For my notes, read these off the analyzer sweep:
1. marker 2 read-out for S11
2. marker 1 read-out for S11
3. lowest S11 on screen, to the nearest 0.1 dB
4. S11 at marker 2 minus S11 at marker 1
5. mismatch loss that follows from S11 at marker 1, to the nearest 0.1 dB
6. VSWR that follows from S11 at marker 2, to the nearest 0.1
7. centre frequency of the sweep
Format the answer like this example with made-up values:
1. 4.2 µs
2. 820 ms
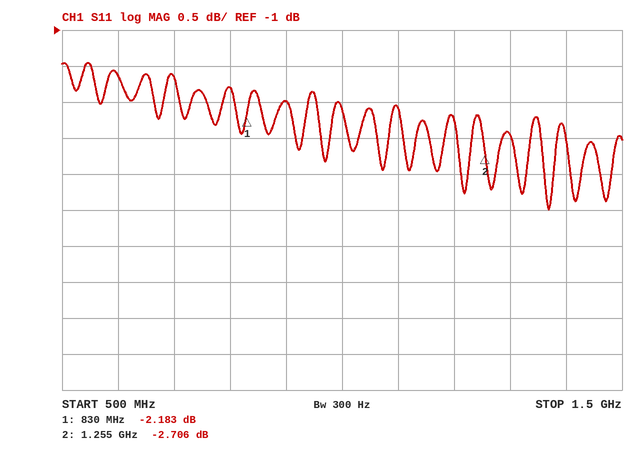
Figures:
1. -2.706 dB
2. -2.183 dB
3. -3.5 dB
4. -0.523 dB
5. 4.0 dB
6. 6.5
7. 1 GHz
